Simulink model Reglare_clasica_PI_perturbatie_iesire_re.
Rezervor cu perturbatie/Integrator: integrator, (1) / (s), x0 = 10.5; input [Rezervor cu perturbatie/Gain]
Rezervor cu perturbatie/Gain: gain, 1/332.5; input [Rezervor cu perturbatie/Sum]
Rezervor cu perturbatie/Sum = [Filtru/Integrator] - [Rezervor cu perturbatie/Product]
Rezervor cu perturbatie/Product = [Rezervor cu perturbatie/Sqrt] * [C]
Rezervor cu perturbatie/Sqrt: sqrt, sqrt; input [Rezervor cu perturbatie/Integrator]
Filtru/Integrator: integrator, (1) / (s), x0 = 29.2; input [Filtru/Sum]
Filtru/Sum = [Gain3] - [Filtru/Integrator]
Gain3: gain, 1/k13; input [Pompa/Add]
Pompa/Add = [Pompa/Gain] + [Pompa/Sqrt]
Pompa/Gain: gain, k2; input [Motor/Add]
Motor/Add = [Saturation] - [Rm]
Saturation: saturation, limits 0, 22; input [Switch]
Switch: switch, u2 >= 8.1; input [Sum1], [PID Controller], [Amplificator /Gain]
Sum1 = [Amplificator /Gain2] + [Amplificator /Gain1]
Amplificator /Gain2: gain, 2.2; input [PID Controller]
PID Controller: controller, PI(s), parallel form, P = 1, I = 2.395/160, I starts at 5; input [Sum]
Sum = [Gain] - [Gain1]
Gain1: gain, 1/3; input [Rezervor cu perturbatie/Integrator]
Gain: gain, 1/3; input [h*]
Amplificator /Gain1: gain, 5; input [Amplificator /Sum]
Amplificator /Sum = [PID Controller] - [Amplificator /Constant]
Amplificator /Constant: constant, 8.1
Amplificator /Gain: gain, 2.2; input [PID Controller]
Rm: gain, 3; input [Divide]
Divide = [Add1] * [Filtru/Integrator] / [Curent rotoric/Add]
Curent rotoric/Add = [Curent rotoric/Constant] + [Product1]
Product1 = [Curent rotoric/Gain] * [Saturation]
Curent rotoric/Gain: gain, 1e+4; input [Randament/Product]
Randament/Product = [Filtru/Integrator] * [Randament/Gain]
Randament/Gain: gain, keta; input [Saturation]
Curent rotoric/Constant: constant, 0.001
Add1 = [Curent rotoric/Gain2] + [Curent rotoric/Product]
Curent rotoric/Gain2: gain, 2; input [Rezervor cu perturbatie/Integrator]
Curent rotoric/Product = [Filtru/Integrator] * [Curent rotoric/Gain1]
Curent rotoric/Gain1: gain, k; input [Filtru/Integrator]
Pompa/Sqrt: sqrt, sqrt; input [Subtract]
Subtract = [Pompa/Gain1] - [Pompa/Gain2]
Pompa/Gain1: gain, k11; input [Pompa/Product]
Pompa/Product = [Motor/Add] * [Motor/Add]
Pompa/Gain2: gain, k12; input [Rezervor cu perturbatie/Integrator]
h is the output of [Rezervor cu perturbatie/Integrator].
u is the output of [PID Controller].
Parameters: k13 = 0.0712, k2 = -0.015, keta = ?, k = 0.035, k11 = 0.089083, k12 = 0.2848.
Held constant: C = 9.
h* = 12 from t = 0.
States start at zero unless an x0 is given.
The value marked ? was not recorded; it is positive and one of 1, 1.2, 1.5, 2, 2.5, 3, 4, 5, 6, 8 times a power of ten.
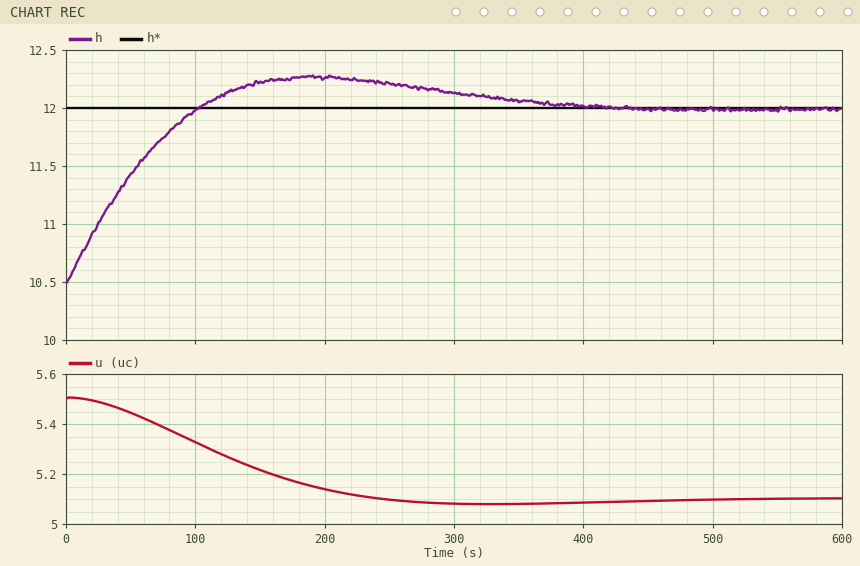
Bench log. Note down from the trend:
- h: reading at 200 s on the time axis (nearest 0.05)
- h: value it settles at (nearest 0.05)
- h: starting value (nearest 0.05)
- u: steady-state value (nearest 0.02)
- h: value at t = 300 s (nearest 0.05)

12.25
12.00
10.50
5.10
12.15
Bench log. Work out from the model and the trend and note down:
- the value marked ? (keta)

0.00012
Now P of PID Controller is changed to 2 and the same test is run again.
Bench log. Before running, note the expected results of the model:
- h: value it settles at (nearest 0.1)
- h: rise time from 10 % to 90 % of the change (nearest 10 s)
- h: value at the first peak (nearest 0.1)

12.0
60 s
12.1
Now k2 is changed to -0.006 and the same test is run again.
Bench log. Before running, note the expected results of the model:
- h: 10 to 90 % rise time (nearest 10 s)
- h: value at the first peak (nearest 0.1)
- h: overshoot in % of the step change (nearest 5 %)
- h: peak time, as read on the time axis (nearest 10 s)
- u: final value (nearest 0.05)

70 s
12.3
20 %
170 s
5.00
